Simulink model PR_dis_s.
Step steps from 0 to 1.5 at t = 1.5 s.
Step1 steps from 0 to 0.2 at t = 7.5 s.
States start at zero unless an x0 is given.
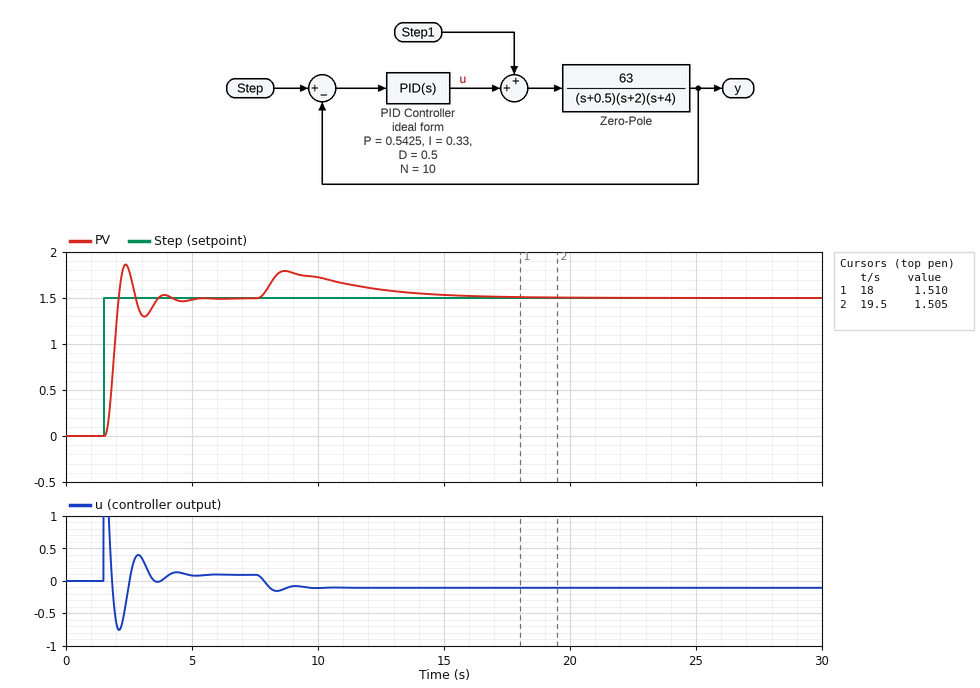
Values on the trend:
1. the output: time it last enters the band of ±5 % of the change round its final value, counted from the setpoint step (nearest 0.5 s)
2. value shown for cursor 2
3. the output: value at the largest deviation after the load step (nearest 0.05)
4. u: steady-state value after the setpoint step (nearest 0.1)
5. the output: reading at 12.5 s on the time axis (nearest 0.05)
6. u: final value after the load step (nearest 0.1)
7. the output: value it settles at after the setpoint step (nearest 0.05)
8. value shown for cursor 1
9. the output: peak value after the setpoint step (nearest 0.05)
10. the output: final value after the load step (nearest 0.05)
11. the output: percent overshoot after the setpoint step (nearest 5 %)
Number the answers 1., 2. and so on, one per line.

1. 2.0 s
2. 1.505
3. 1.80
4. 0.1
5. 1.60
6. -0.1
7. 1.50
8. 1.510
9. 1.85
10. 1.50
11. 25 %
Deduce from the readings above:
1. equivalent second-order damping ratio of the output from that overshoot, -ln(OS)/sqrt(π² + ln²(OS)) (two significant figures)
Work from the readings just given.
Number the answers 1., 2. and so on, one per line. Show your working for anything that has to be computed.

1. ln(0.25) = -1.386; 1.386 / sqrt(9.870 + 1.922) = 0.40
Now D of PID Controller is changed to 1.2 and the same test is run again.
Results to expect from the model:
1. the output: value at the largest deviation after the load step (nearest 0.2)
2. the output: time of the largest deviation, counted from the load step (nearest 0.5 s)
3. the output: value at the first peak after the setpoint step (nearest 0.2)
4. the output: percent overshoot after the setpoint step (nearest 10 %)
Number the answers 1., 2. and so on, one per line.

1. 1.8
2. 2.0 s
3. 2.0
4. 40 %
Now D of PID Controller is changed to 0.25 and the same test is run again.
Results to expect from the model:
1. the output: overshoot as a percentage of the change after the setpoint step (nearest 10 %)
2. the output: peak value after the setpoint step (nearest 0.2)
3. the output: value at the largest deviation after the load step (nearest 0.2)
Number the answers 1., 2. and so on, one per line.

1. 30 %
2. 2.0
3. 1.8
